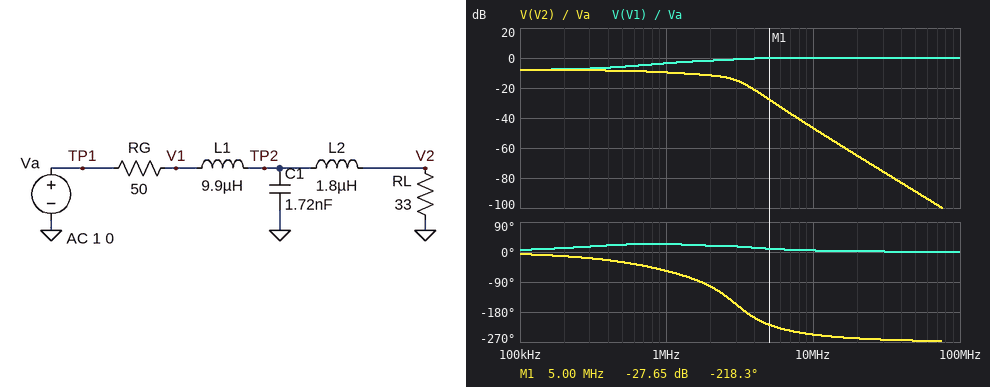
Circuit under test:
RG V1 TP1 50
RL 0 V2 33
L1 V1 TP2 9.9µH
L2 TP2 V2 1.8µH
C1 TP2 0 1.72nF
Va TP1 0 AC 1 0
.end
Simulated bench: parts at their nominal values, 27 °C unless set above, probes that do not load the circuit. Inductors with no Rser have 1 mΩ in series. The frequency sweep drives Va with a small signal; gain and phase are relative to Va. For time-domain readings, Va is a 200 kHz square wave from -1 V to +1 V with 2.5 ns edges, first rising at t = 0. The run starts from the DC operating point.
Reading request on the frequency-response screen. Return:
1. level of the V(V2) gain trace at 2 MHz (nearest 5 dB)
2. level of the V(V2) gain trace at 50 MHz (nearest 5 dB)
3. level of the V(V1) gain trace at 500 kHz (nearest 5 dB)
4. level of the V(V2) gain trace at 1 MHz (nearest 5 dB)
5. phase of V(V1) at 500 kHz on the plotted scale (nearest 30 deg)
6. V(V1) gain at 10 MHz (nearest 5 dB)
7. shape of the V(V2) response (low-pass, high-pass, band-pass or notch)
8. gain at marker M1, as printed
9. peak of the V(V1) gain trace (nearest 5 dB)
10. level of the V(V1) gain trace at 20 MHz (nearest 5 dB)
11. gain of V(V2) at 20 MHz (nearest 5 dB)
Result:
-10 dB
-90 dB
-5 dB
-10 dB
30 deg
0 dB
low-pass
-27.65 dB
0 dB
0 dB
-65 dB
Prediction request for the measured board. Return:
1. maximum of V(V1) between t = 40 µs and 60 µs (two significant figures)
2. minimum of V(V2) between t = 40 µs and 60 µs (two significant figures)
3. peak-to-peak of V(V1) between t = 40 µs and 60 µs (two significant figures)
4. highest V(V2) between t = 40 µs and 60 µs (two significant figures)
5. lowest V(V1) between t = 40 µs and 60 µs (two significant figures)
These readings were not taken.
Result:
1.6 V
-400 mV
3.2 V
400 mV
-1.6 V
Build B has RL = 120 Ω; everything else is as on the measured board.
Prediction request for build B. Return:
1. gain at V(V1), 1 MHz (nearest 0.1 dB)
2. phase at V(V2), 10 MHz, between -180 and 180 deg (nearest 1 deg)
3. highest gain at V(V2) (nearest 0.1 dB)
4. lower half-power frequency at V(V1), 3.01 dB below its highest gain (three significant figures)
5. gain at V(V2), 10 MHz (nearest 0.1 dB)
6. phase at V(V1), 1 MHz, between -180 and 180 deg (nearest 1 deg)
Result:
-6.1 dB
144 deg
-2.2 dB
1.78 MHz
-38.9 dB
2 deg
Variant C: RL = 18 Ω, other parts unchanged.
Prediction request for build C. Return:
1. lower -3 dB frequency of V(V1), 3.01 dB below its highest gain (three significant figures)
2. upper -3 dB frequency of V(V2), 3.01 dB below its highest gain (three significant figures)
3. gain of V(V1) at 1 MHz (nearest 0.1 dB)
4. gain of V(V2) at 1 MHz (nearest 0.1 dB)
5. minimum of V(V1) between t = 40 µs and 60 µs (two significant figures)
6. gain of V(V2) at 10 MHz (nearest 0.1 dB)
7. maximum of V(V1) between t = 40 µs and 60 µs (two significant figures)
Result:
923 kHz
1.20 MHz
-2.7 dB
-14.0 dB
-1.7 V
-51.8 dB
1.7 V
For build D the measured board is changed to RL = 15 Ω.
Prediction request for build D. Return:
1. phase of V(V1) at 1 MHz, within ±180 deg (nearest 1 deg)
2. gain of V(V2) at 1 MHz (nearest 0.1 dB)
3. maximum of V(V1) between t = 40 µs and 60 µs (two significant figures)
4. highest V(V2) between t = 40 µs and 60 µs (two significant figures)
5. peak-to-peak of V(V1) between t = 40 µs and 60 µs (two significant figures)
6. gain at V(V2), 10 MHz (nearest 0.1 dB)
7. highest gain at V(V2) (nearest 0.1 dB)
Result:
29 deg
-15.4 dB
1.8 V
230 mV
3.5 V
-53.3 dB
-12.7 dB
